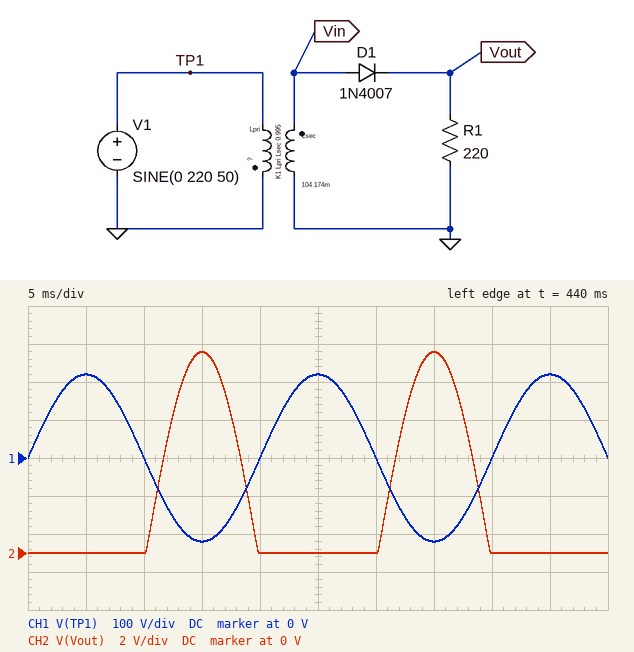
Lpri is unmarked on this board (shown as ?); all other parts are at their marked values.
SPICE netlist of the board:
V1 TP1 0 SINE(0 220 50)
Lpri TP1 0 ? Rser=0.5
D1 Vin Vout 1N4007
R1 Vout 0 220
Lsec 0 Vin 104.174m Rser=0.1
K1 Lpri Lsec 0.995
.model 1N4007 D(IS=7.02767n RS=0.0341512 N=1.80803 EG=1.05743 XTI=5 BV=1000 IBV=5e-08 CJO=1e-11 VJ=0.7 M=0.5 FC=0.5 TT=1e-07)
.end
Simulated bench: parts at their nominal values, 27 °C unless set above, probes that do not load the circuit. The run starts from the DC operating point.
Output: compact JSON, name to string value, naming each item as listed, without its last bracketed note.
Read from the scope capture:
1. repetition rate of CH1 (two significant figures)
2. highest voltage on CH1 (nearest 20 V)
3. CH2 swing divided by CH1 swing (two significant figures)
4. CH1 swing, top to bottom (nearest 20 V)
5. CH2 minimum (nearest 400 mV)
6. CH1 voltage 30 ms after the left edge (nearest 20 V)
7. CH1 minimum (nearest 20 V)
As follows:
{"repetition rate of CH1": "50 Hz", "highest voltage on CH1": "220 V", "CH2 swing divided by CH1 swing": "0.024", "CH1 swing, top to bottom": "440 V", "CH2 minimum": "0 V", "CH1 voltage 30 ms after the left edge": "0 V", "CH1 minimum": "-220 V"}
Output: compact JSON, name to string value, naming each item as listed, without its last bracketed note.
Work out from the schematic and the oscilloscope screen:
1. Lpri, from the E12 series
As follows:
{"Lpri, from the E12 series": "39 H"}
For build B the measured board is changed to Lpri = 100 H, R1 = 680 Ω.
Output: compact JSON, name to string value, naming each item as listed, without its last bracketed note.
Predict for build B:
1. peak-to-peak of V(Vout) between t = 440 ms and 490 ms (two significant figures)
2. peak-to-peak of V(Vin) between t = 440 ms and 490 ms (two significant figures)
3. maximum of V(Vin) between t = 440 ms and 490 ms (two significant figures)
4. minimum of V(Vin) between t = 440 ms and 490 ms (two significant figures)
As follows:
{"peak-to-peak of V(Vout) between t = 440 ms and 490 ms": "6.4 V", "peak-to-peak of V(Vin) between t = 440 ms and 490 ms": "14 V", "maximum of V(Vin) between t = 440 ms and 490 ms": "7.1 V", "minimum of V(Vin) between t = 440 ms and 490 ms": "-7.1 V"}
